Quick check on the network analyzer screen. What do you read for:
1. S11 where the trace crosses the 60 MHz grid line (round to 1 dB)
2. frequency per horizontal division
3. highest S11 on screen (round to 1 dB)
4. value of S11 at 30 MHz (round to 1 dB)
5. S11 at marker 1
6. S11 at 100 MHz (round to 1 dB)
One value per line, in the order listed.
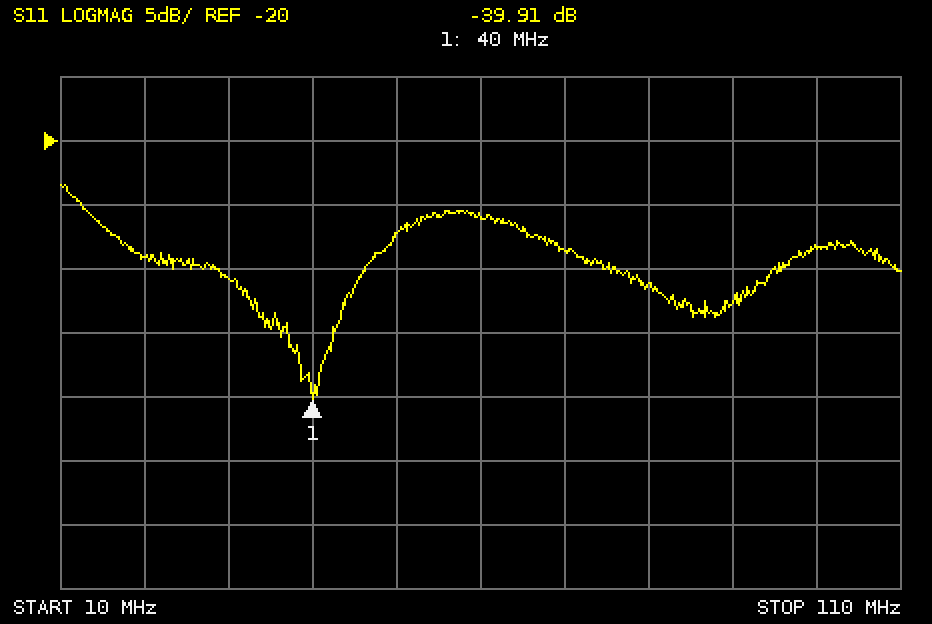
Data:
-26 dB
10 MHz
-23 dB
-31 dB
-39.91 dB
-28 dB
